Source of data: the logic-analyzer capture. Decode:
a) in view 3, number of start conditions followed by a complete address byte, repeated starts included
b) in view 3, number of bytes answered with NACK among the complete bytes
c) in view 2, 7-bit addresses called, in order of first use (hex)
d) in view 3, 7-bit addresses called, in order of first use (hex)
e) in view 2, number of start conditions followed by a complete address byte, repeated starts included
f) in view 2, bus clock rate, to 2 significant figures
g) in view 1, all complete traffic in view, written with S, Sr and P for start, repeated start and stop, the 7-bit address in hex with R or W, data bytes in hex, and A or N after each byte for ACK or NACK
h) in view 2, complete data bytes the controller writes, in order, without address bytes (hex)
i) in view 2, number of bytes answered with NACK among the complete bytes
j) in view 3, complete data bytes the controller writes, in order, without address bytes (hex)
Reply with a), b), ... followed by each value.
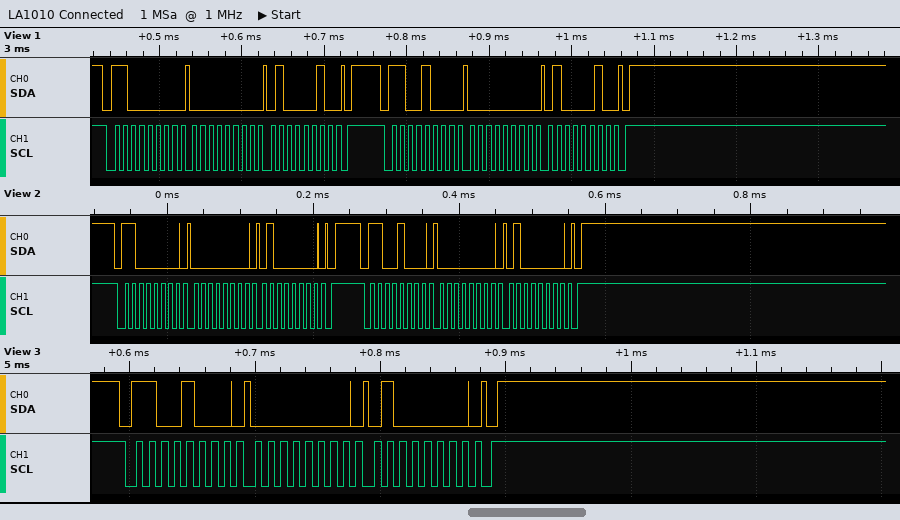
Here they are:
a) 1
b) 0
c) 0x60 0x64
d) 0x64
e) 2
f) 100 kHz
g) S 60W A 00 A 42 A P S 64W A 00 A 42 A P
h) 00 40 00 40
i) 0
j) 00 40
